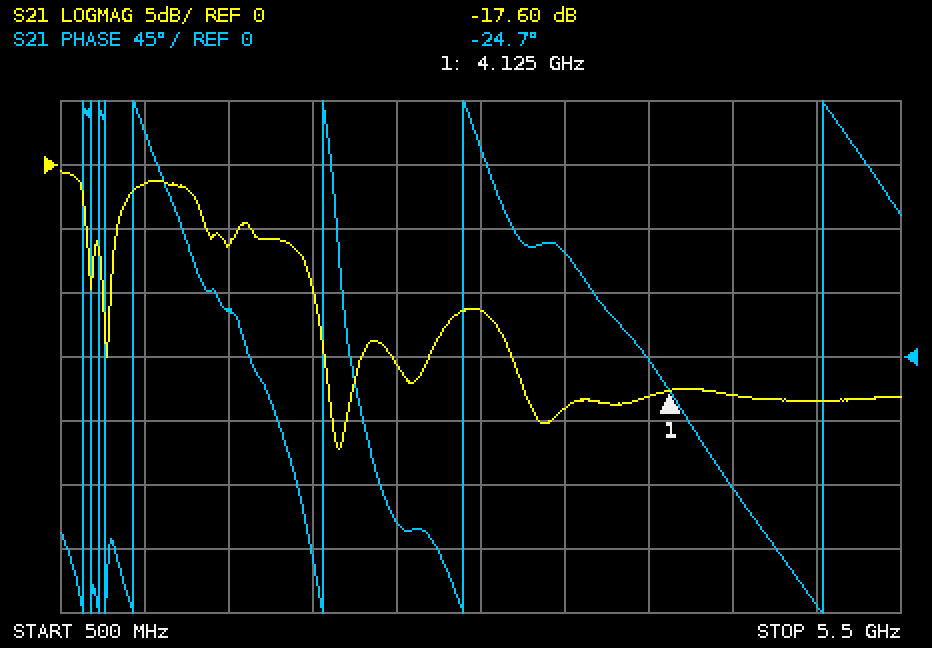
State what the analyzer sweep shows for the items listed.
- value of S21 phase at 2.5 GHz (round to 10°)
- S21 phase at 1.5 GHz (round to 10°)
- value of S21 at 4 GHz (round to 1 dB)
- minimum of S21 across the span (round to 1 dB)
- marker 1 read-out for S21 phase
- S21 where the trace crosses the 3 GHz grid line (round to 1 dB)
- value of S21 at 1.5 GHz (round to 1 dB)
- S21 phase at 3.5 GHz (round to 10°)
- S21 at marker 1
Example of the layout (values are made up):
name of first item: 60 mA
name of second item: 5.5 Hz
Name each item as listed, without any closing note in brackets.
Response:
value of S21 phase at 2.5 GHz: -120°
S21 phase at 1.5 GHz: 30°
value of S21 at 4 GHz: -18 dB
minimum of S21 across the span: -22 dB
marker 1 read-out for S21 phase: -24.7°
S21 where the trace crosses the 3 GHz grid line: -11 dB
value of S21 at 1.5 GHz: -6 dB
S21 phase at 3.5 GHz: 70°
S21 at marker 1: -17.60 dB
